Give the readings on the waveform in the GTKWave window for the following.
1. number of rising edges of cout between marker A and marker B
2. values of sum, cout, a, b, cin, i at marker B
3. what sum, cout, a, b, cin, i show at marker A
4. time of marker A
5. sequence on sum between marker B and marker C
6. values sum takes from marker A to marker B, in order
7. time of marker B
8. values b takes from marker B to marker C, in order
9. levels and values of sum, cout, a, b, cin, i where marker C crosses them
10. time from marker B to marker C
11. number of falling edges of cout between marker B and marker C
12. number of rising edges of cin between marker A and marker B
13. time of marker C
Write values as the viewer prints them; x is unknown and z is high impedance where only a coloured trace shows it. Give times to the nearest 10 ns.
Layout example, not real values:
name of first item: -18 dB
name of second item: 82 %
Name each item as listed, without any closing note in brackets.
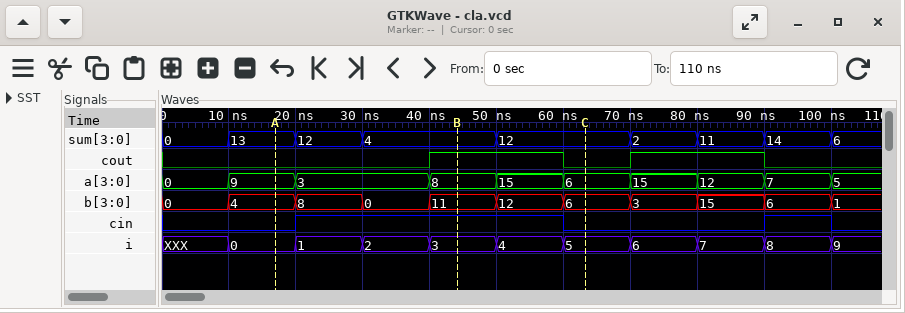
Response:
number of rising edges of cout between marker A and marker B: 1
values of sum, cout, a, b, cin, i at marker B: sum=4, cout=1, a=8, b=11, cin=1, i=3
what sum, cout, a, b, cin, i show at marker A: sum=13, cout=0, a=9, b=4, cin=0, i=0
time of marker A: 20 ns
sequence on sum between marker B and marker C: 4, 12
values sum takes from marker A to marker B, in order: 13, 12, 4
time of marker B: 40 ns
values b takes from marker B to marker C, in order: 11, 12, 6
levels and values of sum, cout, a, b, cin, i where marker C crosses them: sum=12, cout=0, a=6, b=6, cin=0, i=5
time from marker B to marker C: 20 ns
number of falling edges of cout between marker B and marker C: 1
number of rising edges of cin between marker A and marker B: 1
time of marker C: 60 ns
